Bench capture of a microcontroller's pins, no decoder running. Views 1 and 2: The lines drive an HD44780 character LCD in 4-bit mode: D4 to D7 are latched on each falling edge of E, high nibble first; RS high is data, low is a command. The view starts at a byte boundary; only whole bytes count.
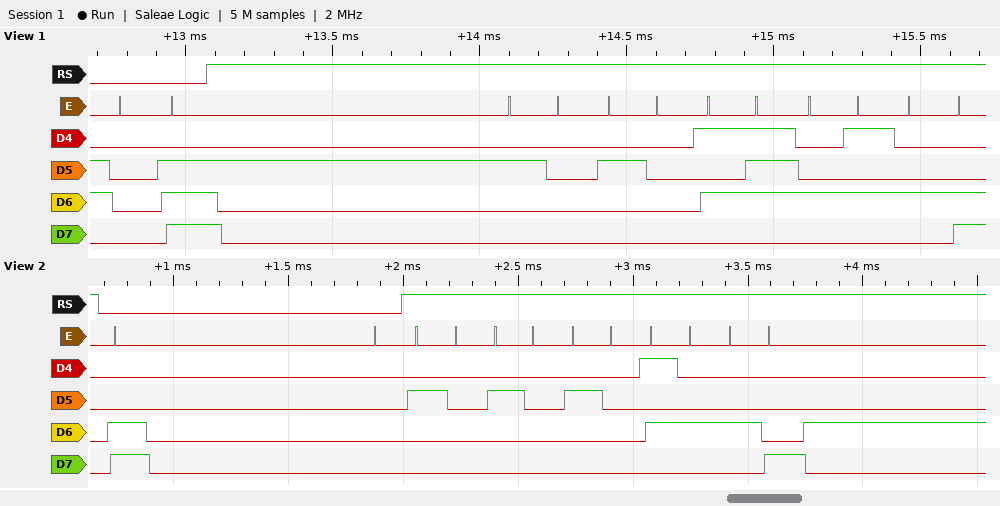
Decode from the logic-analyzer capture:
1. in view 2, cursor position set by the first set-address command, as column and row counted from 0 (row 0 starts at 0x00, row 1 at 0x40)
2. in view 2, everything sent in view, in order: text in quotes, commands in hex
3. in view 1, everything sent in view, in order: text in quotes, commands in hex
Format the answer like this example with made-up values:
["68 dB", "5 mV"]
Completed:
["column 0, row 1", "0xC0 \"   TH\"", "0x0E \"  WEL\""]
